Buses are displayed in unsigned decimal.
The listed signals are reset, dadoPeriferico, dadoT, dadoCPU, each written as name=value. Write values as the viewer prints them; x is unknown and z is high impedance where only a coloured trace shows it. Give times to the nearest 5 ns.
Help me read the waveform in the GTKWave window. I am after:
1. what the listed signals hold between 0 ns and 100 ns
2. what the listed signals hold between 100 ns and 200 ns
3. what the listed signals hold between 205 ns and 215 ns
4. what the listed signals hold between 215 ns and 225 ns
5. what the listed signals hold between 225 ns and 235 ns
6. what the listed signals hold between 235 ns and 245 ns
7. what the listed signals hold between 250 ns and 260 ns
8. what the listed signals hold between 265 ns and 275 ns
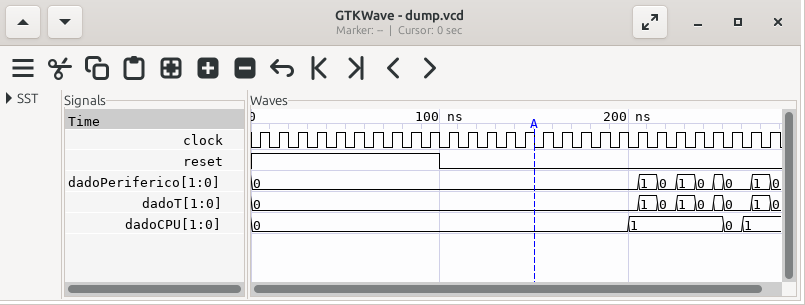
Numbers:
reset=1, dadoPeriferico=0, dadoT=0, dadoCPU=0
reset=0, dadoPeriferico=0, dadoT=0, dadoCPU=0
reset=0, dadoPeriferico=1, dadoT=1, dadoCPU=1
reset=0, dadoPeriferico=0, dadoT=0, dadoCPU=1
reset=0, dadoPeriferico=1, dadoT=1, dadoCPU=1
reset=0, dadoPeriferico=0, dadoT=0, dadoCPU=1
reset=0, dadoPeriferico=0, dadoT=0, dadoCPU=0
reset=0, dadoPeriferico=1, dadoT=1, dadoCPU=1
